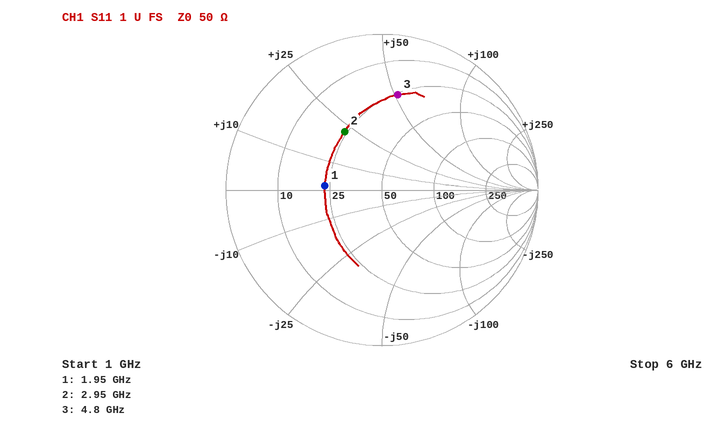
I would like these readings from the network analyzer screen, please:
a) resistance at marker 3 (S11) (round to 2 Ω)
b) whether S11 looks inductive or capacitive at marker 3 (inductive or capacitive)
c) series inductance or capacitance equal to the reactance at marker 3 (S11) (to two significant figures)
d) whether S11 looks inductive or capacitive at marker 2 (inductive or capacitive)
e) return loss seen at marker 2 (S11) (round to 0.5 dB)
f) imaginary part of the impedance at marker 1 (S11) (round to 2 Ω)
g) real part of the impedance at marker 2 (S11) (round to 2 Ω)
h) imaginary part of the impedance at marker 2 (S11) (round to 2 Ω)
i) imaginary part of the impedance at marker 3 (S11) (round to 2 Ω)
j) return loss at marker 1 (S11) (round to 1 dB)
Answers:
26 Ω
inductive
1.7 nH
inductive
7.0 dB
+2 Ω
24 Ω
+22 Ω
+52 Ω
9 dB
